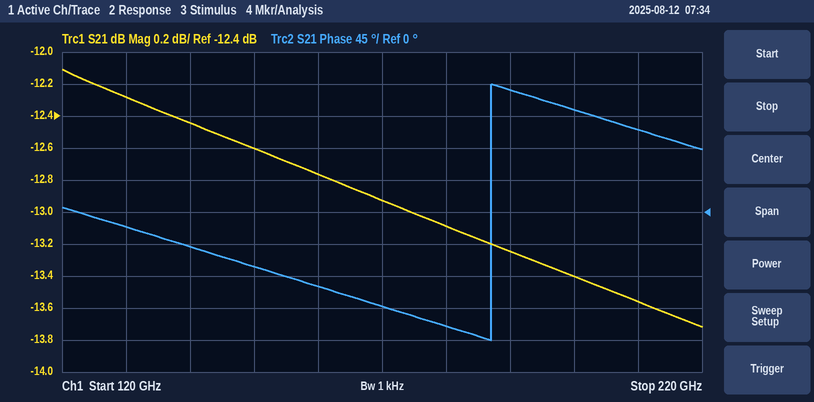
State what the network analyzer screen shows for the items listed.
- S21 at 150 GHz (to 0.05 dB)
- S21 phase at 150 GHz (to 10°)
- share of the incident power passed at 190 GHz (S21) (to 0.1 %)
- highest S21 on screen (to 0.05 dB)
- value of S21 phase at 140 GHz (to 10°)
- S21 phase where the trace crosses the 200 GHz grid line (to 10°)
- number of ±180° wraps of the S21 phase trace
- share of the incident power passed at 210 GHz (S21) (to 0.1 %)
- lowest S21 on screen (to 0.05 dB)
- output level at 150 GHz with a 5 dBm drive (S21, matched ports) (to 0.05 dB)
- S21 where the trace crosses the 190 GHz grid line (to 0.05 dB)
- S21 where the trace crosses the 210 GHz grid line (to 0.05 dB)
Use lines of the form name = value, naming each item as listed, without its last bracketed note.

S21 at 150 GHz = -12.60 dB
S21 phase at 150 GHz = -80°
share of the incident power passed at 190 GHz (S21) = 4.7 %
highest S21 on screen = -12.10 dB
value of S21 phase at 140 GHz = -50°
S21 phase where the trace crosses the 200 GHz grid line = 140°
number of ±180° wraps of the S21 phase trace = 1
share of the incident power passed at 210 GHz (S21) = 4.4 %
lowest S21 on screen = -13.70 dB
output level at 150 GHz with a 5 dBm drive (S21, matched ports) = -7.60 dBm
S21 where the trace crosses the 190 GHz grid line = -13.25 dB
S21 where the trace crosses the 210 GHz grid line = -13.55 dB
